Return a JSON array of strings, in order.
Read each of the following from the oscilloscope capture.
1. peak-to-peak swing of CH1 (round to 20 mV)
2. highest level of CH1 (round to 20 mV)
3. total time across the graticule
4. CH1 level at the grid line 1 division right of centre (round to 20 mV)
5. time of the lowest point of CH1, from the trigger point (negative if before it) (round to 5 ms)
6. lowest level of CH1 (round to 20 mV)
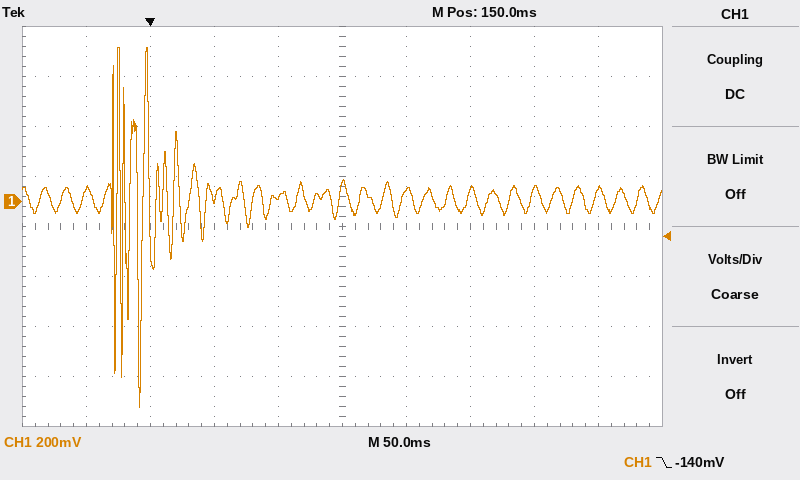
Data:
["1.44 V", "620 mV", "500 ms", "40 mV", "-10 ms", "-820 mV"]
